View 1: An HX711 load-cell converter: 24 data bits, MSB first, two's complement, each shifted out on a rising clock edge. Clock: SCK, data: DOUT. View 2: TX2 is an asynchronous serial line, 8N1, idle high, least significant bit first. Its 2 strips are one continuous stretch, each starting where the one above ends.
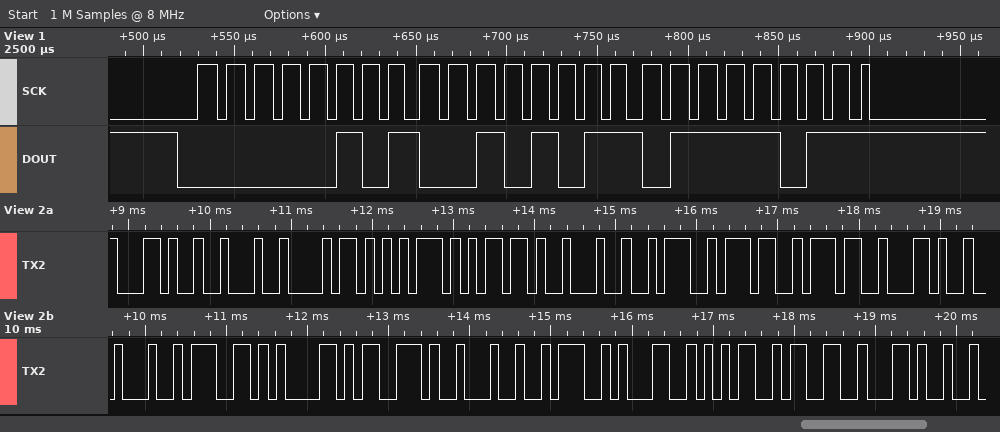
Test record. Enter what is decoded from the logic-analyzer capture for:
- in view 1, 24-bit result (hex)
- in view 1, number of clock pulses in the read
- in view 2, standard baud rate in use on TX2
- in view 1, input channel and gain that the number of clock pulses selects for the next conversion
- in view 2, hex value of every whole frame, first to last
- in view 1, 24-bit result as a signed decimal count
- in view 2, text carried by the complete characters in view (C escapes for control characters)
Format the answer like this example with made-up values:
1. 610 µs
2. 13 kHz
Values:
1. 0x052B7B
2. 25
3. 9600 baud
4. channel A, gain 128
5. 2C 22 68 75 6D 22 3A 37 37 2C 22 67 61 73 22 3A 31 35 33 2C
6. 338811
7. ",\"hum\":77,\"gas\":153,"
